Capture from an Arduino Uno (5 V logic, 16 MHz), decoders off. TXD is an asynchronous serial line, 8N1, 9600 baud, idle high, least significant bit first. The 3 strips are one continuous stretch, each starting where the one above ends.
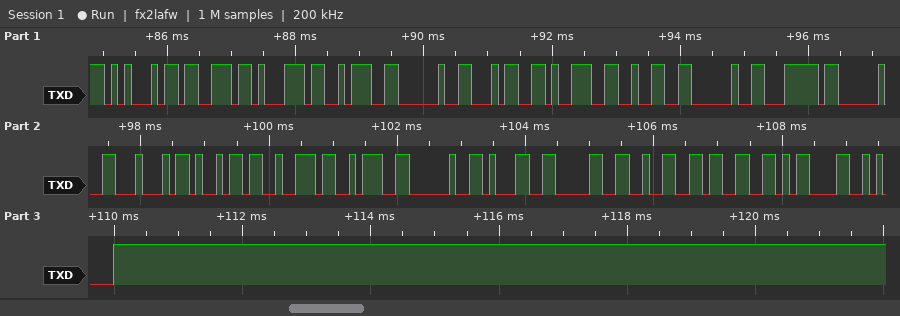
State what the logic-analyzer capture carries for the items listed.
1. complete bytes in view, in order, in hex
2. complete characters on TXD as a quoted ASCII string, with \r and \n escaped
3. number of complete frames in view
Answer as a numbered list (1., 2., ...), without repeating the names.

1. 45 73 71 3A 20 34 39 32 20 7C 20 44 69 72 3A 20 31 30 32 33 0D 0A
2. "Esq: 492 | Dir: 1023\r\n"
3. 22
